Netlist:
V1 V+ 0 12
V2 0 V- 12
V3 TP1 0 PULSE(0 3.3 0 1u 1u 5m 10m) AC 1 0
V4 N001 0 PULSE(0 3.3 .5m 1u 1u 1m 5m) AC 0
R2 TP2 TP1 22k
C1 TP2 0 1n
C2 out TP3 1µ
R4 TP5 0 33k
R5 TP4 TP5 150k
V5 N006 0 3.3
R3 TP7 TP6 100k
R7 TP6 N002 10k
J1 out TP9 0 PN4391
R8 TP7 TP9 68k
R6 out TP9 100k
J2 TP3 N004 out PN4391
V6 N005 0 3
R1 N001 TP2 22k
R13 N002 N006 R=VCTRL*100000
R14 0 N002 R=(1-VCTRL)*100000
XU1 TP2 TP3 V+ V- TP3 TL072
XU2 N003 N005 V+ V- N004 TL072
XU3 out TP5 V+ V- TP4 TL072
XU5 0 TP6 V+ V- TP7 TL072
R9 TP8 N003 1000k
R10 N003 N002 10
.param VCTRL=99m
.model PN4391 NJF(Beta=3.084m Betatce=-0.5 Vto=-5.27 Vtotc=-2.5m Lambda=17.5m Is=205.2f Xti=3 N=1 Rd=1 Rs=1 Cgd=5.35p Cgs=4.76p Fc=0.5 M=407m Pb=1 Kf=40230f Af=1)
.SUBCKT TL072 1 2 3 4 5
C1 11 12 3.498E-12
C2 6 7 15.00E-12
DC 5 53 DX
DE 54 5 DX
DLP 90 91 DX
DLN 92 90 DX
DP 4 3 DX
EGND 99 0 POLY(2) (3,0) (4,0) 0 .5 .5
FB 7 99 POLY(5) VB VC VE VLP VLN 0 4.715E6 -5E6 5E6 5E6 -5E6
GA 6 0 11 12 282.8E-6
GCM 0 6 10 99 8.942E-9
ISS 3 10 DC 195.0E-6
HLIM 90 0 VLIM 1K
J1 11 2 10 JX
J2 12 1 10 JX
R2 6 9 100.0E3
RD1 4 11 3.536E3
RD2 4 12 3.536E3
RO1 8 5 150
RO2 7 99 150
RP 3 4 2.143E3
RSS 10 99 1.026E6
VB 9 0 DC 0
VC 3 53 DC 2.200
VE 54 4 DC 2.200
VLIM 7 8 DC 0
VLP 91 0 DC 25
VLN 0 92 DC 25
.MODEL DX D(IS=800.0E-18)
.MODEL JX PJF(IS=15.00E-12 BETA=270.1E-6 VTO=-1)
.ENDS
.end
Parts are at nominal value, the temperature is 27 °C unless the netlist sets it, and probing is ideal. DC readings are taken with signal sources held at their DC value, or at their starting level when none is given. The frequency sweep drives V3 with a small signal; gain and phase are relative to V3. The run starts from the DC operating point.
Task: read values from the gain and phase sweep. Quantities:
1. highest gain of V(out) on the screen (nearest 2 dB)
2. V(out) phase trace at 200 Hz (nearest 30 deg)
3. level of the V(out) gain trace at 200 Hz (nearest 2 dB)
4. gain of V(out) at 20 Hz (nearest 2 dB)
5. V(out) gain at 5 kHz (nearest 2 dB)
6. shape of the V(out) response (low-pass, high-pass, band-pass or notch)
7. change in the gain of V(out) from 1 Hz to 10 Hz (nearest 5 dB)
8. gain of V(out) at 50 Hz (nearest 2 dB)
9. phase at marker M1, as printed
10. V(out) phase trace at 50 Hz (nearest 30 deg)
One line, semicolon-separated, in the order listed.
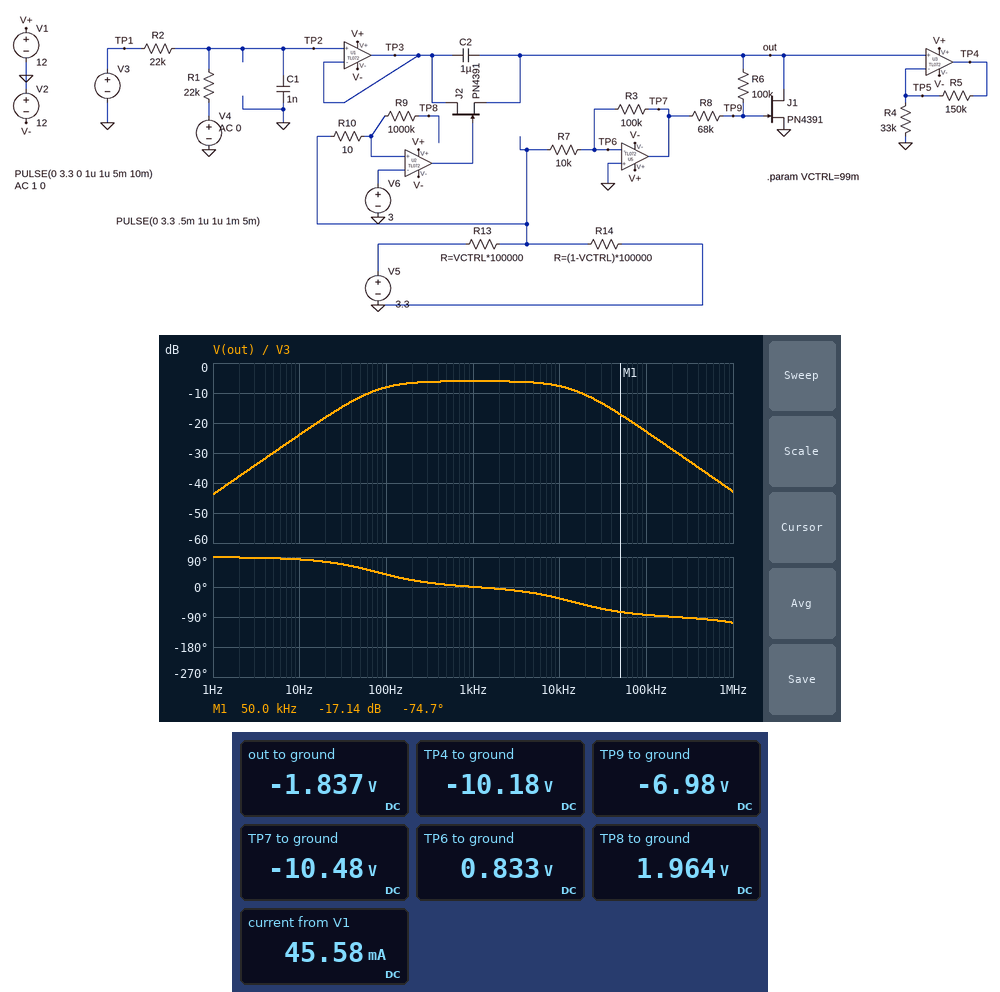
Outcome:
-6 dB; 30 deg; -6 dB; -18 dB; -6 dB; band-pass; 20 dB; -12 dB; -74.7 deg; 60 deg
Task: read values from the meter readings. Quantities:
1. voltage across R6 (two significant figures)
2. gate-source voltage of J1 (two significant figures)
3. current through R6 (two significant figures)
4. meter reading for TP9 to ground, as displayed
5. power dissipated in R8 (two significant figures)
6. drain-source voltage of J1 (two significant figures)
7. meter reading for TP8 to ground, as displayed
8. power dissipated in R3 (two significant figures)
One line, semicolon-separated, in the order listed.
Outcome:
5.1 V; -7.0 V; 51 µA; -6.98 V; 180 µW; -1.8 V; 1.964 V; 1.3 mW
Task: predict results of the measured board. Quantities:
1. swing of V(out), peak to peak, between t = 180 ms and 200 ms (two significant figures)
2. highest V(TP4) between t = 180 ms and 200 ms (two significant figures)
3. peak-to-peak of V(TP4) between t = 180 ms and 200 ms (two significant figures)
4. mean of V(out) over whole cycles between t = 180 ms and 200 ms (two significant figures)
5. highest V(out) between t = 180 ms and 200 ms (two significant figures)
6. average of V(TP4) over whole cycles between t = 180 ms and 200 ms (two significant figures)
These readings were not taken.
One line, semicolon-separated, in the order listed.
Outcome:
3.6 V; 7.7 V; 18 V; -860 mV; 1.4 V; -4.6 V
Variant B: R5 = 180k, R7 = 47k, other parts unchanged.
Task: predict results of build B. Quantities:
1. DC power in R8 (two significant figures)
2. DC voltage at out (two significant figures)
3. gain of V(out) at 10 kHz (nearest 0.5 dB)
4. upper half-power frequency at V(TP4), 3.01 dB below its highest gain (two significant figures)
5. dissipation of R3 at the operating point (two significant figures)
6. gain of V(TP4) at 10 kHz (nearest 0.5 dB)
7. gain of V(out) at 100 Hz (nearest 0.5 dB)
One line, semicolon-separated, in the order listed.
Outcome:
68 µW; -2.5 mV; -8.0 dB; 18 kHz; 280 µW; 8.5 dB; -32.0 dB
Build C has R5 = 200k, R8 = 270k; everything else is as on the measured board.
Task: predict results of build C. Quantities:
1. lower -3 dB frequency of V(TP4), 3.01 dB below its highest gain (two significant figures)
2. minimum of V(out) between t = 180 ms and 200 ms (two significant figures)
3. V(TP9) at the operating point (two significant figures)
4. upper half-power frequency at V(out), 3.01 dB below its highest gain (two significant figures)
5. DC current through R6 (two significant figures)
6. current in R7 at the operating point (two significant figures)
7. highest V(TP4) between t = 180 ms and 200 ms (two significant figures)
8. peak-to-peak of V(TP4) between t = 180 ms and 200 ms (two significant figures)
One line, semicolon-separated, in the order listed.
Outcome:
1.8 kHz; -1.2 V; -2.8 V; 19 kHz; 28 µA; 110 µA; 8.0 V; 16 V
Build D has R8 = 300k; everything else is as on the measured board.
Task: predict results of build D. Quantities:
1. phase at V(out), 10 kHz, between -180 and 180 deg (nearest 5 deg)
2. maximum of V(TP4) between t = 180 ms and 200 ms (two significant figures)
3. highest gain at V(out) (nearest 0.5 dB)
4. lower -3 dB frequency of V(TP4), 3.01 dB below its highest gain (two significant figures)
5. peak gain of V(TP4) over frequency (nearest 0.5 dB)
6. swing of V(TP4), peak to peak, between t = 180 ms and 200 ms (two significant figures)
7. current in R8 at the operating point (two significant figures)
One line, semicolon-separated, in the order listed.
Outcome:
-20 deg; 6.2 V; -7.5 dB; 1.9 kHz; 7.5 dB; 13 V; 26 µA
